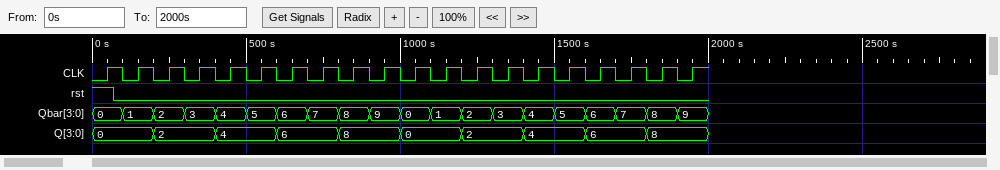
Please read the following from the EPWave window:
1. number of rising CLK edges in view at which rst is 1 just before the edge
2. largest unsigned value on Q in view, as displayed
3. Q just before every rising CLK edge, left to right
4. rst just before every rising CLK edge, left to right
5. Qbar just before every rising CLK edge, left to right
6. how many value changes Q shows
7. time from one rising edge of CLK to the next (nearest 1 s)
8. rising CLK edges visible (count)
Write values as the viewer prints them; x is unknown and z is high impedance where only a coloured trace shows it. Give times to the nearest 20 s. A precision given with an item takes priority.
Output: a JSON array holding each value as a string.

["1", "8", "0, 0, 2, 2, 4, 4, 6, 6, 8, 8, 0, 0, 2, 2, 4, 4, 6, 6, 8, 8", "1 0 0 0 0 0 0 0 0 0 0 0 0 0 0 0 0 0 0 0", "0, 1, 2, 3, 4, 5, 6, 7, 8, 9, 0, 1, 2, 3, 4, 5, 6, 7, 8, 9", "9", "100 s", "20"]
